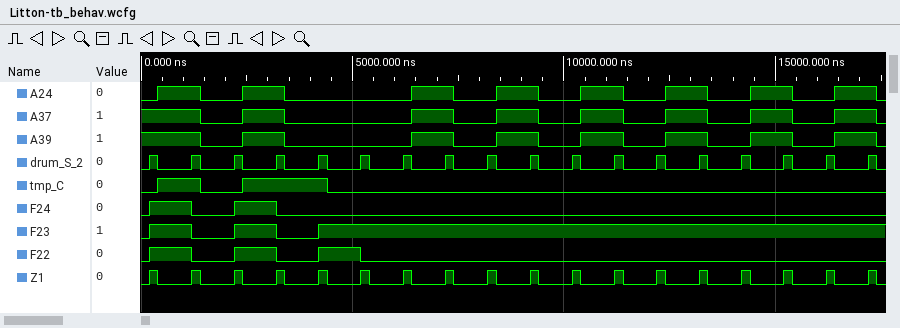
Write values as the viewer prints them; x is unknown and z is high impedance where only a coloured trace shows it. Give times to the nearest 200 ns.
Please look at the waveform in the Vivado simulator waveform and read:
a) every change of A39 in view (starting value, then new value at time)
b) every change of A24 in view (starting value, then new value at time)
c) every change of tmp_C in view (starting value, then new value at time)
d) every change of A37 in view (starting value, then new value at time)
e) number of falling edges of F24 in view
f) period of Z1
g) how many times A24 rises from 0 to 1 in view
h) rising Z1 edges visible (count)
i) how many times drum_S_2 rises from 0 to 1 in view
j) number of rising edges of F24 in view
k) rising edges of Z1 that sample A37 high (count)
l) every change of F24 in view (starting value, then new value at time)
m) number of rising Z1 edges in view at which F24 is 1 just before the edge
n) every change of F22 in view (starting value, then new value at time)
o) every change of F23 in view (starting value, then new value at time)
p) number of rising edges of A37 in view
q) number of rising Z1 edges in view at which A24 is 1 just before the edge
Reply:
1, 0 at 1400 ns, 1 at 2400 ns, 0 at 3400 ns, 1 at 6400 ns, 0 at 7400 ns, 1 at 8400 ns, 0 at 9400 ns, 1 at 10400 ns, 0 at 11400 ns, 1 at 12400 ns, 0 at 13400 ns, 1 at 14400 ns, 0 at 15400 ns, 1 at 16400 ns, 0 at 17400 ns
0, 1 at 400 ns, 0 at 1400 ns, 1 at 2400 ns, 0 at 3400 ns, 1 at 6400 ns, 0 at 7400 ns, 1 at 8400 ns, 0 at 9400 ns, 1 at 10400 ns, 0 at 11400 ns, 1 at 12400 ns, 0 at 13400 ns, 1 at 14400 ns, 0 at 15400 ns, 1 at 16400 ns, 0 at 17400 ns
0, 1 at 400 ns, 0 at 1400 ns, 1 at 2400 ns, 0 at 4400 ns
1, 0 at 1400 ns, 1 at 2400 ns, 0 at 3400 ns, 1 at 6400 ns, 0 at 7400 ns, 1 at 8400 ns, 0 at 9400 ns, 1 at 10400 ns, 0 at 11400 ns, 1 at 12400 ns, 0 at 13400 ns, 1 at 14400 ns, 0 at 15400 ns, 1 at 16400 ns, 0 at 17400 ns
2
1000 ns
8
18
18
2
9
0, 1 at 200 ns, 0 at 1200 ns, 1 at 2200 ns, 0 at 3200 ns
2
0, 1 at 200 ns, 0 at 1200 ns, 1 at 2200 ns, 0 at 3200 ns, 1 at 4200 ns, 0 at 5200 ns
0, 1 at 200 ns, 0 at 1200 ns, 1 at 2200 ns, 0 at 3200 ns, 1 at 4200 ns
7
8
